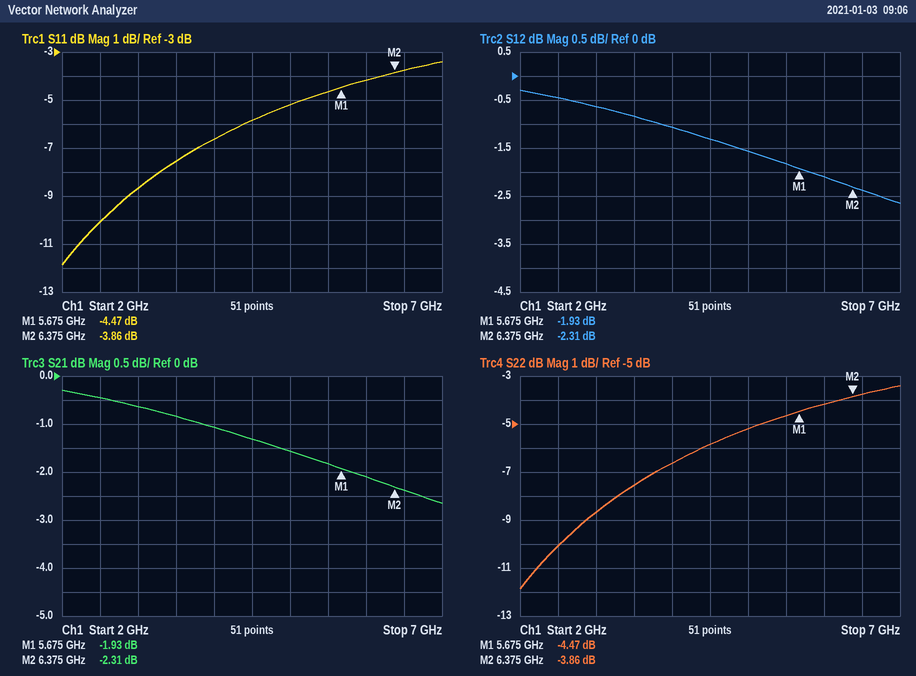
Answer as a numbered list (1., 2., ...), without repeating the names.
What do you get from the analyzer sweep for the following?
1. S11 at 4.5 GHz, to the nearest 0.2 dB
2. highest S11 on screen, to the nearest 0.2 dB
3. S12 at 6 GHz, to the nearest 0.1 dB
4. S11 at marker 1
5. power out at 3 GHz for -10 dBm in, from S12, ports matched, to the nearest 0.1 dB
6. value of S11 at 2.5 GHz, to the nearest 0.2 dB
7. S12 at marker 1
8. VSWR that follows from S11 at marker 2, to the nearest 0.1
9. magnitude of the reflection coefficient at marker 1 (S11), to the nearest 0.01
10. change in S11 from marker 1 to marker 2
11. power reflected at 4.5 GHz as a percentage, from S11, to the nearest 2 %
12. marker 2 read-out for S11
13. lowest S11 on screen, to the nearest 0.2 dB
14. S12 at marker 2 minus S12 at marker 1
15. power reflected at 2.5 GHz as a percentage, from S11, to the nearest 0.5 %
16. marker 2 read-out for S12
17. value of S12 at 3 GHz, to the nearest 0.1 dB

1. -5.8 dB
2. -3.4 dB
3. -2.1 dB
4. -4.47 dB
5. -10.6 dBm
6. -10.0 dB
7. -1.93 dB
8. 4.6
9. 0.60
10. 0.61 dB
11. 26 %
12. -3.86 dB
13. -11.8 dB
14. -0.38 dB
15. 10.0 %
16. -2.31 dB
17. -0.6 dB
